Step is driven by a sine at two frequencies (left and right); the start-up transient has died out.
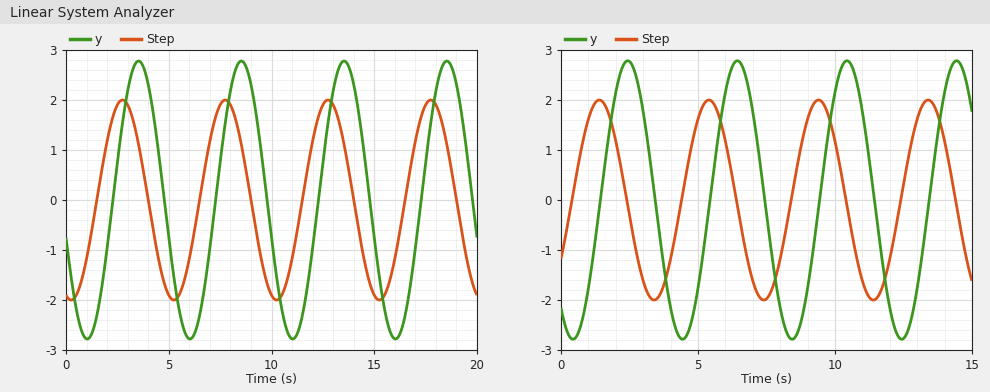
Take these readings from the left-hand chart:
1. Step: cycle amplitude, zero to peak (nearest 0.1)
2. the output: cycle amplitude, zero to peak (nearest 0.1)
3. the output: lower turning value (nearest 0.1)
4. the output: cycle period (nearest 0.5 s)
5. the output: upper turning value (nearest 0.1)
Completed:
2.0
2.8
-2.8
5.0 s
2.8
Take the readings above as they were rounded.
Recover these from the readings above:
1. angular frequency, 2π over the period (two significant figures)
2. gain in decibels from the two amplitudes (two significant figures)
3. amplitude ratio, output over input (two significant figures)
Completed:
1.3 rad/s
2.9 dB
1.4
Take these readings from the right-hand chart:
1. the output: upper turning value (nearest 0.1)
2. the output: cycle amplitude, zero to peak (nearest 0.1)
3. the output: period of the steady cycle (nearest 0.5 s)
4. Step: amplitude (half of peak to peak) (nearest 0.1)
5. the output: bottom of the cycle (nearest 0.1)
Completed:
2.8
2.8
4.0 s
2.0
-2.8
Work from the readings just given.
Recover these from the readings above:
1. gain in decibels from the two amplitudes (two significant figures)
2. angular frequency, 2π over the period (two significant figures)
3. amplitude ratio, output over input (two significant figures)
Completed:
2.9 dB
1.6 rad/s
1.4
